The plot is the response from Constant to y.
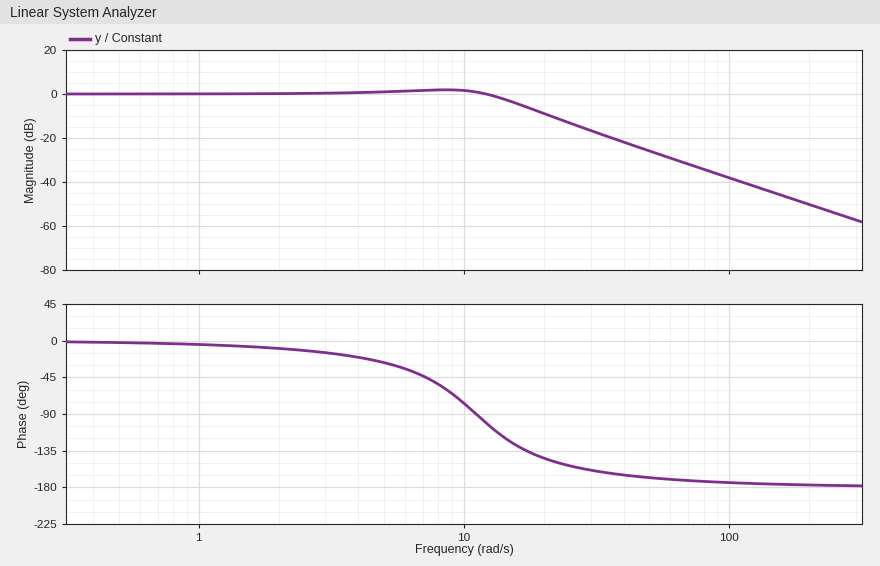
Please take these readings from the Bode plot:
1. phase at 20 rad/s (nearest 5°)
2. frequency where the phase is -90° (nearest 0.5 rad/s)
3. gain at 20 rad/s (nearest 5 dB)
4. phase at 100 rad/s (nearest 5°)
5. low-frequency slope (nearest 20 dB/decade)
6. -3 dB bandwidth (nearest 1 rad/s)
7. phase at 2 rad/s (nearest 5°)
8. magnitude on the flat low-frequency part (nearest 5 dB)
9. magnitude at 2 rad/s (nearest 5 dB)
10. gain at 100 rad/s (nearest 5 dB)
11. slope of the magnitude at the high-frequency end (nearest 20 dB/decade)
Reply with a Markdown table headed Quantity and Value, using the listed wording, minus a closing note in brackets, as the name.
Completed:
| Quantity | Value |
|---|---|
| phase at 20 rad/s | -145° |
| frequency where the phase is -90° | 11.0 rad/s |
| gain at 20 rad/s | -10 dB |
| phase at 100 rad/s | -175° |
| low-frequency slope | 0 dB/decade |
| -3 dB bandwidth | 15 rad/s |
| phase at 2 rad/s | -10° |
| magnitude on the flat low-frequency part | 0 dB |
| magnitude at 2 rad/s | 0 dB |
| gain at 100 rad/s | -40 dB |
| slope of the magnitude at the high-frequency end | -40 dB/decade |
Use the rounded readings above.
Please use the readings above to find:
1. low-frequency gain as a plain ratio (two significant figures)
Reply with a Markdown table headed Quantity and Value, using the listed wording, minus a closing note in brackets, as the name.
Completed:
| Quantity | Value |
|---|---|
| low-frequency gain as a plain ratio | 1.0 |
